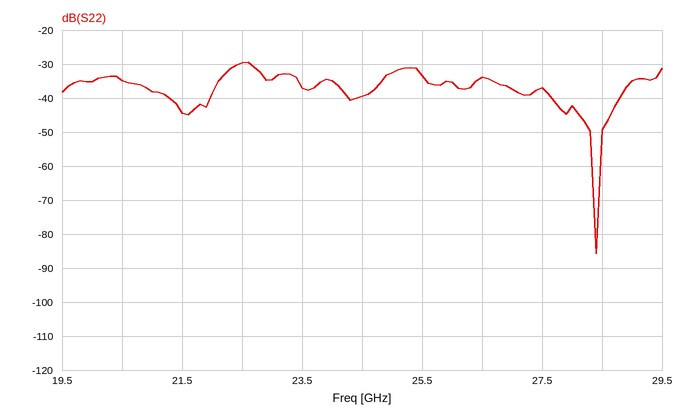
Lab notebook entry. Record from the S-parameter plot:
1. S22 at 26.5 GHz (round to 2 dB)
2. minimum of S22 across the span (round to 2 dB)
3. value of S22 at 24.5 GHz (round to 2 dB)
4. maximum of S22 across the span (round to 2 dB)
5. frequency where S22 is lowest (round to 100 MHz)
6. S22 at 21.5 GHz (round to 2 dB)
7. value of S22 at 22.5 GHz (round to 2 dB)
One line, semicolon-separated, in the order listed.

-34 dB; -86 dB; -40 dB; -30 dB; 28.4 GHz; -44 dB; -30 dB
